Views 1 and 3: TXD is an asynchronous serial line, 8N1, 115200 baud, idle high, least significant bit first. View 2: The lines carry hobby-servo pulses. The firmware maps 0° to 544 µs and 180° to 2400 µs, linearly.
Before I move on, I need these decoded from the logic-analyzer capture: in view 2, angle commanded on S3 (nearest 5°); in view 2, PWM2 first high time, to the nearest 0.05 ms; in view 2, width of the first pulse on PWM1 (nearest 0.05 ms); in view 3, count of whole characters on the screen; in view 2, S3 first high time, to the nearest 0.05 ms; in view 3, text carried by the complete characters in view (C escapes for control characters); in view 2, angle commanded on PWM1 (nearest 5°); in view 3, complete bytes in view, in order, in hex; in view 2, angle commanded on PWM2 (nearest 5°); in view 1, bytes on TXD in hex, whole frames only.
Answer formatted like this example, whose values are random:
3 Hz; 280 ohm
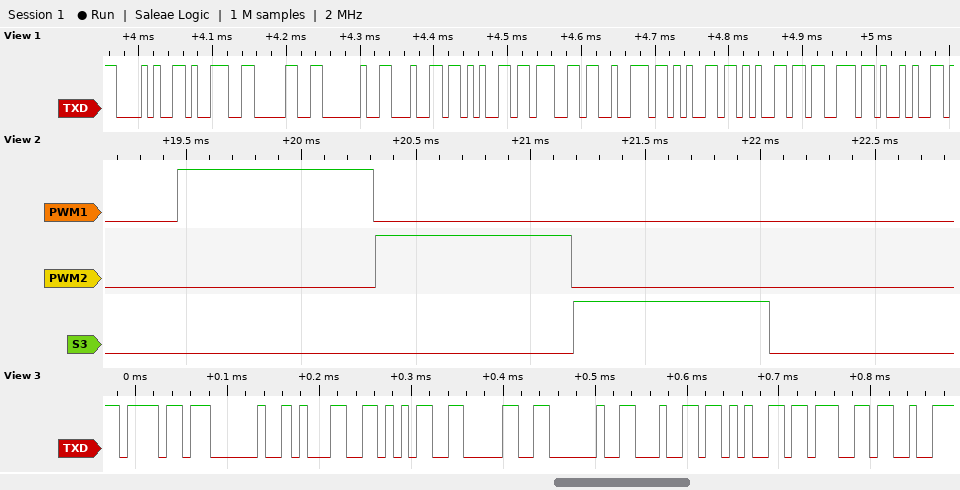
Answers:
30°; 0.85 ms; 0.85 ms; 9; 0.85 ms; "o 150 deg"; 30°; 0x6F 0x20 0x31 0x35 0x30 0x20 0x64 0x65 0x67; 30°; 28 39 30 20 64 65 67 72 65 65 73 29
